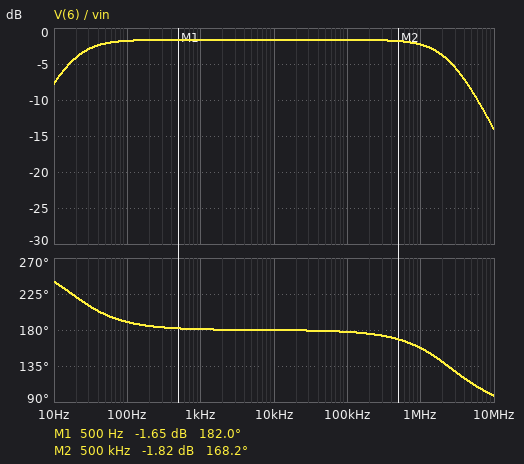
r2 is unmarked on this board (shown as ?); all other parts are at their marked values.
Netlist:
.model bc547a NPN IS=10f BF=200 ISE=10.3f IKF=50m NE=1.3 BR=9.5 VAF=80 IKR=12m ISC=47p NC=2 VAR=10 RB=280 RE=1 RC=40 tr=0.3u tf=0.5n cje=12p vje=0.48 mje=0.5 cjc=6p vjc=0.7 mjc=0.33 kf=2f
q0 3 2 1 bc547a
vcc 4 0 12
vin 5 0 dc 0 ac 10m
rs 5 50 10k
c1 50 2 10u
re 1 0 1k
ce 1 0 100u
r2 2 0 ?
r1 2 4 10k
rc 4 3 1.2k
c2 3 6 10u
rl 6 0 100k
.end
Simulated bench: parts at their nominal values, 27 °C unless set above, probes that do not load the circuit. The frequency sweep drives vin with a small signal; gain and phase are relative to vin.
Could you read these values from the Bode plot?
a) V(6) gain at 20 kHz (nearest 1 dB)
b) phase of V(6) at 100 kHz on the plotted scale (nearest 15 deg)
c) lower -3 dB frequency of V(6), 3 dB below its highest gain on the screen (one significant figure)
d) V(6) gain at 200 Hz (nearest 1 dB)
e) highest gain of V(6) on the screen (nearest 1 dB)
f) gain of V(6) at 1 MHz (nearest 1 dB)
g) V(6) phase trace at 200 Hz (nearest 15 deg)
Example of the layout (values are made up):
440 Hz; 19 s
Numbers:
-2 dB; 180 deg; 20 Hz; -2 dB; -2 dB; -2 dB; 180 deg
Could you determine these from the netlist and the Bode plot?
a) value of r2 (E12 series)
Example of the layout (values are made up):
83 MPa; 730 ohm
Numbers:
820 Ω
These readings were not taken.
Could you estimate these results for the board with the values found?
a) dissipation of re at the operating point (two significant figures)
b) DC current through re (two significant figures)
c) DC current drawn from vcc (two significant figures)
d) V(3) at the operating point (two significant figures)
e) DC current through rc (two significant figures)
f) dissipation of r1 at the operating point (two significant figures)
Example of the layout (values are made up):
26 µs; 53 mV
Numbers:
82 µW; 290 µA; 1.4 mA; 12 V; 280 µA; 12 mW
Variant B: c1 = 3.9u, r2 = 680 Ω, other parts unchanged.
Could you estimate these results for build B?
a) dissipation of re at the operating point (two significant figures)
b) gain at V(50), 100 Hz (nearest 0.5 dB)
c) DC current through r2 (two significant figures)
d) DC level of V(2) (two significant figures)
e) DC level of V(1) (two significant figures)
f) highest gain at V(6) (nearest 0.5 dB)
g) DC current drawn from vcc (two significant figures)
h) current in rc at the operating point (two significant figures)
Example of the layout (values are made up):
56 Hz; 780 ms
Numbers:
25 µW; -23.0 dB; 1.1 mA; 760 mV; 160 mV; -8.0 dB; 1.3 mA; 160 µA
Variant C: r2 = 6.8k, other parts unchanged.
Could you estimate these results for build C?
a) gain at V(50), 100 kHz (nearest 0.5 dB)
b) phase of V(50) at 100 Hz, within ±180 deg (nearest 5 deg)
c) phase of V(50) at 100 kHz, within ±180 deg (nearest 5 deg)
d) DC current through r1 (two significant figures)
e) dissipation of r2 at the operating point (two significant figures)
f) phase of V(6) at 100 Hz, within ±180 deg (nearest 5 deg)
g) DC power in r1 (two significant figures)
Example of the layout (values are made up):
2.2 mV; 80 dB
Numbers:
-21.5 dB; -35 deg; -10 deg; 730 µA; 3.3 mW; -155 deg; 5.3 mW
